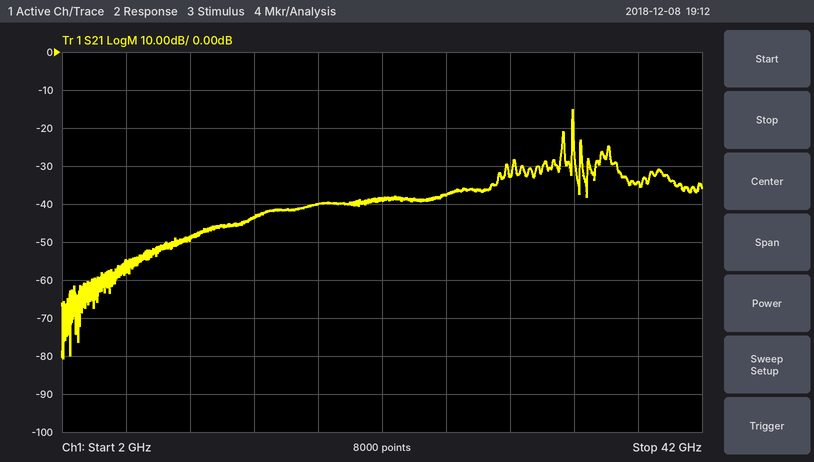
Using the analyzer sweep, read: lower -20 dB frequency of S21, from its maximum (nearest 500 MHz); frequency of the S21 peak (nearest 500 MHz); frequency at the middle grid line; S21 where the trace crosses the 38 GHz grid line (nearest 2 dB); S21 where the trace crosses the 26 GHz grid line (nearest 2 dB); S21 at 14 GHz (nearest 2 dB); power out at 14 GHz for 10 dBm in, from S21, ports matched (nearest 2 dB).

29.0 GHz
34.0 GHz
22 GHz
-34 dB
-38 dB
-44 dB
-34 dBm
